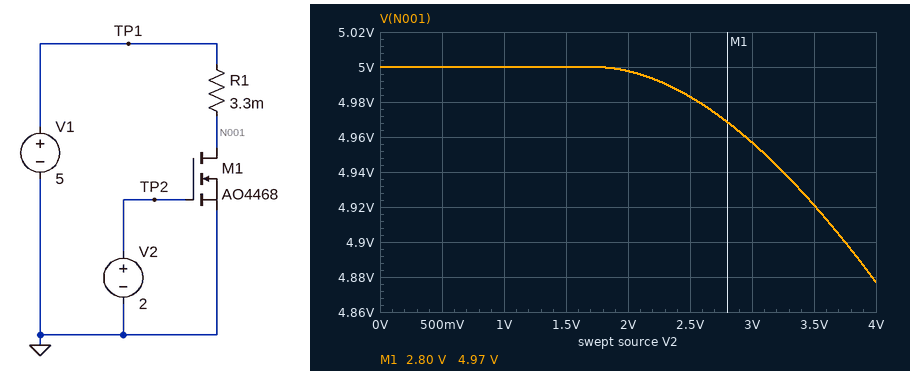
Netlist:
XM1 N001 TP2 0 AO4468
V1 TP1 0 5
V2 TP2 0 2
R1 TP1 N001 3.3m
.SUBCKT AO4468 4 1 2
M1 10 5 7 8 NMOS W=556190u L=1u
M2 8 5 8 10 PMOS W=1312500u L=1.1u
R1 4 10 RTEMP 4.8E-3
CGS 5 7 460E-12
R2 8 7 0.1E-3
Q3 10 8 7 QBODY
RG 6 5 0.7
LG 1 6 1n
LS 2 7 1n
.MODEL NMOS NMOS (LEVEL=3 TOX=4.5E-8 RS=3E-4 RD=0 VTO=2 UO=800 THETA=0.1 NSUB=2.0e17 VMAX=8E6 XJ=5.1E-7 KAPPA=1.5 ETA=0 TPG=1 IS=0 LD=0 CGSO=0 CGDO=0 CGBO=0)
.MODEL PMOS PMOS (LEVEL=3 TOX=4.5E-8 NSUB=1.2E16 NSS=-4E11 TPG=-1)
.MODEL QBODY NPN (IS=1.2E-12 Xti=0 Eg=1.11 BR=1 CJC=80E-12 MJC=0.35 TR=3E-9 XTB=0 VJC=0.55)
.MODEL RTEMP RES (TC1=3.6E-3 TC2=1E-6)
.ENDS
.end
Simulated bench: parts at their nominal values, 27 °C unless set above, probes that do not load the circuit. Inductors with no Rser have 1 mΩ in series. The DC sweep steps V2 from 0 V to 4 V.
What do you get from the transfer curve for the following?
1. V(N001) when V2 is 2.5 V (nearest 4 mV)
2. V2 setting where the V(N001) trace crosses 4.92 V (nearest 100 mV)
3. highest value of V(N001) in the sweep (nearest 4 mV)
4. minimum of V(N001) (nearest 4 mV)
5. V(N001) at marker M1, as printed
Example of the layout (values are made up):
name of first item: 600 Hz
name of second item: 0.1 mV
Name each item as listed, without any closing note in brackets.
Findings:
V(N001) when V2 is 2.5 V: 4.984 V
V2 setting where the V(N001) trace crosses 4.92 V: 3.5 V
highest value of V(N001) in the sweep: 5.000 V
minimum of V(N001): 4.876 V
V(N001) at marker M1, as printed: 4.97 V
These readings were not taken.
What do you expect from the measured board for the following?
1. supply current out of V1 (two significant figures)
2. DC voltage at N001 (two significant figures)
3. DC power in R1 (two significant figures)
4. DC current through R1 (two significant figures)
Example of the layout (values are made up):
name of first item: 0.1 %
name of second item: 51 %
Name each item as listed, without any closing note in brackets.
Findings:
supply current out of V1: 710 mA
DC voltage at N001: 5.0 V
DC power in R1: 1.7 mW
DC current through R1: 710 mA
